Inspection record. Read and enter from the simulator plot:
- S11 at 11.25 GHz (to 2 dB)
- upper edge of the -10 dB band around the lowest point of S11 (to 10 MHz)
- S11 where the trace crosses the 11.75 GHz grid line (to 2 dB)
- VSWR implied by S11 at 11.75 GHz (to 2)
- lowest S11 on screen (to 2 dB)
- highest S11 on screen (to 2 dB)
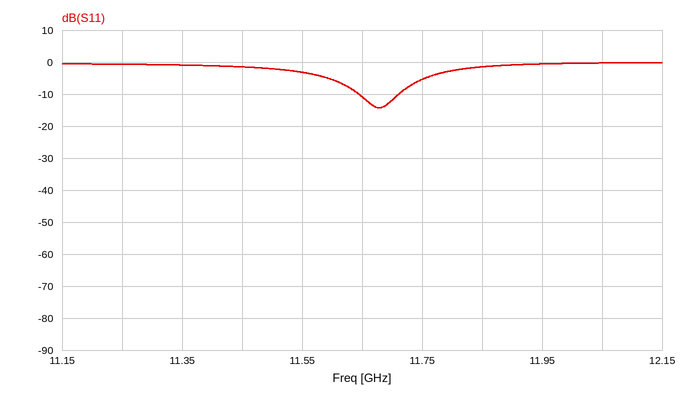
0 dB
11.71 GHz
-6 dB
4
-14 dB
0 dB
